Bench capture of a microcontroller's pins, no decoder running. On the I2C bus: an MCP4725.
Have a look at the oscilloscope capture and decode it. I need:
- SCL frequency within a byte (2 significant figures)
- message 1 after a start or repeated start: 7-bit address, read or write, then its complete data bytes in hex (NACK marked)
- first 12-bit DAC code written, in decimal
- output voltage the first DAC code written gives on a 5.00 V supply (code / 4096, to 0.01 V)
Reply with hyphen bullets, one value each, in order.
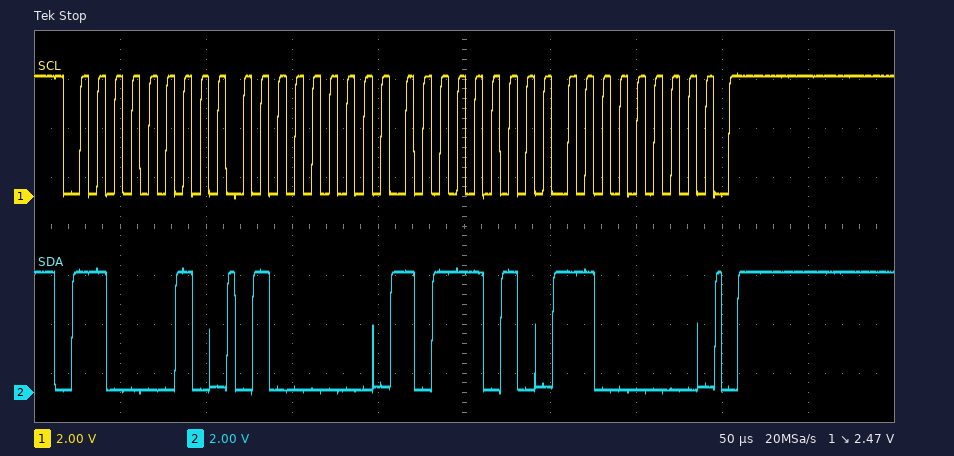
- 100 kHz
- 0x61 write: 40 BA C0
- 2988
- 3.65 V
